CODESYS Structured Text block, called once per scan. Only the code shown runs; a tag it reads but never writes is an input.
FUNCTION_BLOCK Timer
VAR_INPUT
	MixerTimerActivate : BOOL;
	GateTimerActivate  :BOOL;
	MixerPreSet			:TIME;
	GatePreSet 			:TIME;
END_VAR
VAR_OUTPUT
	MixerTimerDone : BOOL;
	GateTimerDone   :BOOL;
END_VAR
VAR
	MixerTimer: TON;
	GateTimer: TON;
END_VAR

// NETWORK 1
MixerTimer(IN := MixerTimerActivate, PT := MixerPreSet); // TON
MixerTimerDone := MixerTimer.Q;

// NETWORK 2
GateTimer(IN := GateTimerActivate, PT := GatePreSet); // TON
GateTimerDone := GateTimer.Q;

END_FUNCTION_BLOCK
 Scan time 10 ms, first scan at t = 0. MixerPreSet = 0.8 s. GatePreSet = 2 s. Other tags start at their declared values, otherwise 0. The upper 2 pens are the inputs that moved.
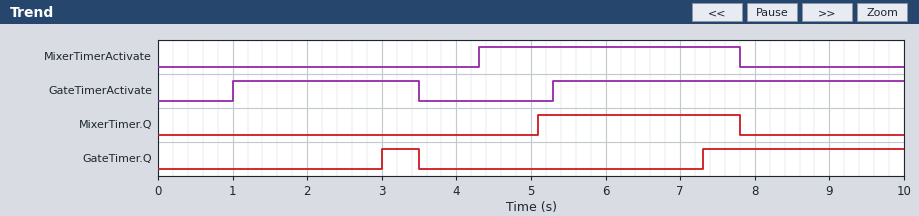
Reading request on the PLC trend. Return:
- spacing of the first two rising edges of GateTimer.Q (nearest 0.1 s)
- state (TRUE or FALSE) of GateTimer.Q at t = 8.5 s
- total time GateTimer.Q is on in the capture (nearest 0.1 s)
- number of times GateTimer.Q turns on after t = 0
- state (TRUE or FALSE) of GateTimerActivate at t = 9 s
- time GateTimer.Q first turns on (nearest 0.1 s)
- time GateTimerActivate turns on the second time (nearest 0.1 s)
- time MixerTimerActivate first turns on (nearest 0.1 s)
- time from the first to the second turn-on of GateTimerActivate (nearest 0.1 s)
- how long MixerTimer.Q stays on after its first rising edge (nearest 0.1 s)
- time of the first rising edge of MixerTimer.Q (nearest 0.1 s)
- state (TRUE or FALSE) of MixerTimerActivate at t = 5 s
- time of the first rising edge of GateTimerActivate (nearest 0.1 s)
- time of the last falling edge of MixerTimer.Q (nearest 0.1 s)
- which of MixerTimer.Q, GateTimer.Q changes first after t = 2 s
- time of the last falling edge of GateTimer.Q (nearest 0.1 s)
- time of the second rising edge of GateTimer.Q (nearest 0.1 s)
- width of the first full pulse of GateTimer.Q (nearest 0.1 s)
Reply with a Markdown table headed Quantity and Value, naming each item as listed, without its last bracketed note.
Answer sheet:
| Quantity | Value |
|---|---|
| spacing of the first two rising edges of GateTimer.Q | 4.3 s |
| state (TRUE or FALSE) of GateTimer.Q at t = 8.5 s | TRUE |
| total time GateTimer.Q is on in the capture | 3.2 s |
| number of times GateTimer.Q turns on after t = 0 | 2 |
| state (TRUE or FALSE) of GateTimerActivate at t = 9 s | TRUE |
| time GateTimer.Q first turns on | 3.0 s |
| time GateTimerActivate turns on the second time | 5.3 s |
| time MixerTimerActivate first turns on | 4.3 s |
| time from the first to the second turn-on of GateTimerActivate | 4.3 s |
| how long MixerTimer.Q stays on after its first rising edge | 2.7 s |
| time of the first rising edge of MixerTimer.Q | 5.1 s |
| state (TRUE or FALSE) of MixerTimerActivate at t = 5 s | TRUE |
| time of the first rising edge of GateTimerActivate | 1.0 s |
| time of the last falling edge of MixerTimer.Q | 7.8 s |
| which of MixerTimer.Q, GateTimer.Q changes first after t = 2 s | GateTimer.Q |
| time of the last falling edge of GateTimer.Q | 3.5 s |
| time of the second rising edge of GateTimer.Q | 7.3 s |
| width of the first full pulse of GateTimer.Q | 0.5 s |
